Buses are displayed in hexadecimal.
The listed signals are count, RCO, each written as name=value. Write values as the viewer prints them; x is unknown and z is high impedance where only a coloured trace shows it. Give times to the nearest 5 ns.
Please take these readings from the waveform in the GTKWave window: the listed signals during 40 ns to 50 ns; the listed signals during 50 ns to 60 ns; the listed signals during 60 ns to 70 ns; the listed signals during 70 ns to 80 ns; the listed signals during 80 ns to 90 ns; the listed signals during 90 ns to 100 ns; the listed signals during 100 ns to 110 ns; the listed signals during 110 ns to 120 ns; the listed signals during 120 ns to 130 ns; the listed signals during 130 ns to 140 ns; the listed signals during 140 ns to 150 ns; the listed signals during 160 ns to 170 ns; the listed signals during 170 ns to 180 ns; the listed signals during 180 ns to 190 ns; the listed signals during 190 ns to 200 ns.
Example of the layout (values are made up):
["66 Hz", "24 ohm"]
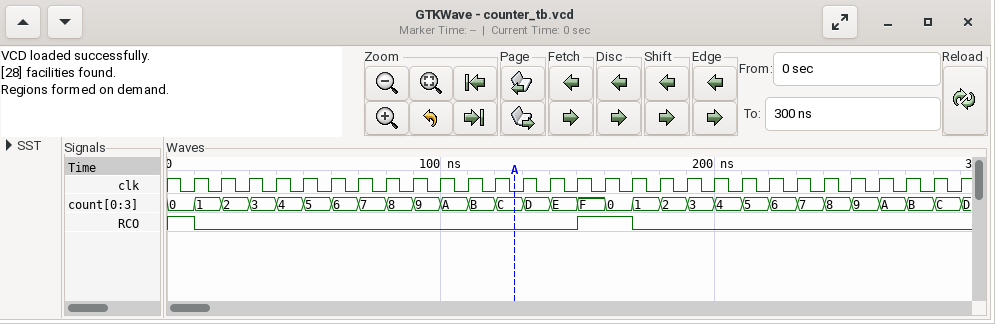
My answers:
["count=4, RCO=0", "count=5, RCO=0", "count=6, RCO=0", "count=7, RCO=0", "count=8, RCO=0", "count=9, RCO=0", "count=A, RCO=0", "count=B, RCO=0", "count=C, RCO=0", "count=D, RCO=0", "count=E, RCO=0", "count=0, RCO=1", "count=1, RCO=0", "count=2, RCO=0", "count=3, RCO=0"]
